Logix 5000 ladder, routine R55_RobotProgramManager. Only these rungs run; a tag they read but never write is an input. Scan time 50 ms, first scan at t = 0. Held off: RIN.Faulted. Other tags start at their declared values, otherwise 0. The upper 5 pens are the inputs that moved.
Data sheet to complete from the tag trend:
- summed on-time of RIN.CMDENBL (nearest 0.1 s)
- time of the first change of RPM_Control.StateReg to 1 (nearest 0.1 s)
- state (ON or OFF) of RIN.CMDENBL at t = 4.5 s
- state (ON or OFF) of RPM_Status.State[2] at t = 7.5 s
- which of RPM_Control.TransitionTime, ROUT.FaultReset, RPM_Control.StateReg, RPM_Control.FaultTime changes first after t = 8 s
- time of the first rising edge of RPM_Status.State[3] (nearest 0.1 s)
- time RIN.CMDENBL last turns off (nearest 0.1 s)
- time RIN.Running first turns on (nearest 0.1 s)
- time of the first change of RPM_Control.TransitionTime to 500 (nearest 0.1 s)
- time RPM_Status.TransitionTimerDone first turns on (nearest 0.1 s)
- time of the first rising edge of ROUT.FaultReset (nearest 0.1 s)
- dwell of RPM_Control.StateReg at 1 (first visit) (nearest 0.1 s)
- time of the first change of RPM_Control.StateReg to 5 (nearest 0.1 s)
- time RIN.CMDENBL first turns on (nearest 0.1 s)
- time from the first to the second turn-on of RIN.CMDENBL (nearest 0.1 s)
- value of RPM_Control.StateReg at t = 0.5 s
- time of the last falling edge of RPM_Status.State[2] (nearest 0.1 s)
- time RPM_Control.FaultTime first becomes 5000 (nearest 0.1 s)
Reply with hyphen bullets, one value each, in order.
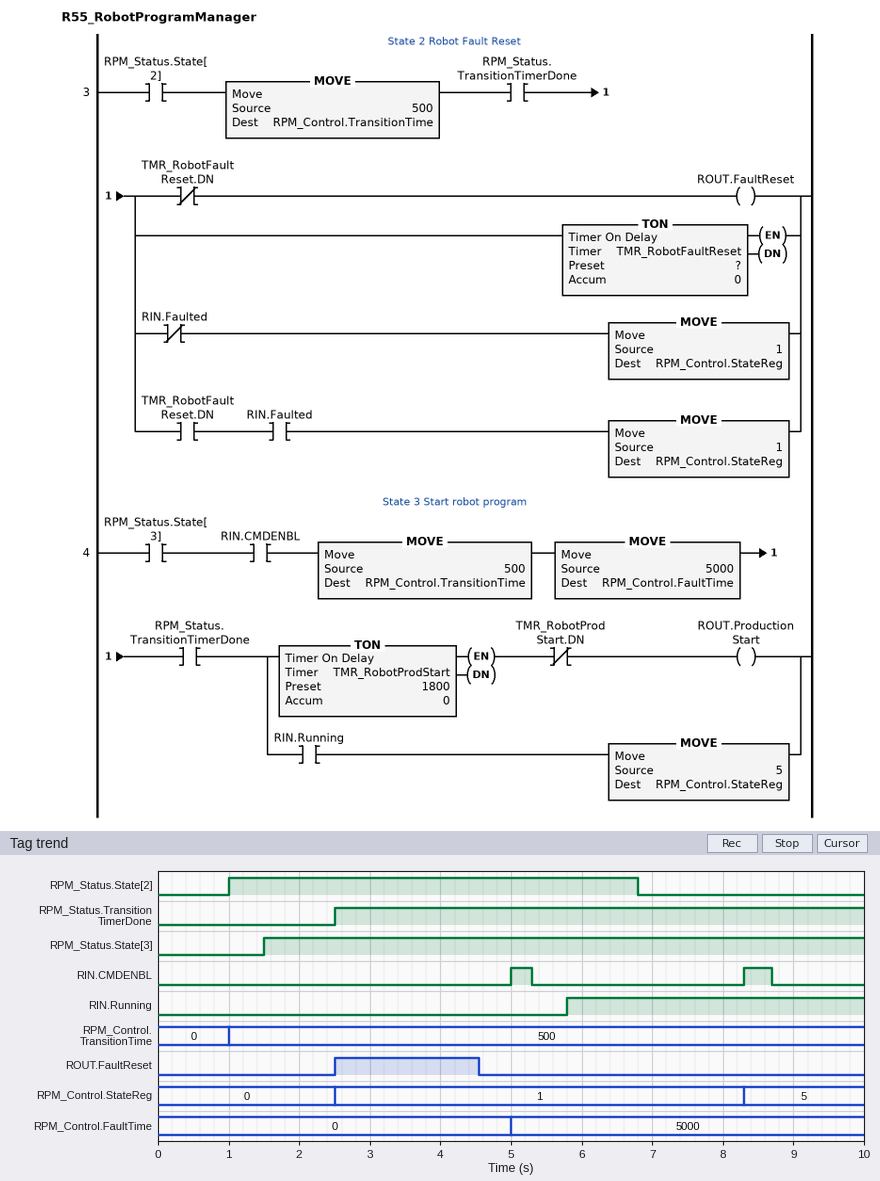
- 0.7 s
- 2.5 s
- OFF
- OFF
- RPM_Control.StateReg
- 1.5 s
- 8.7 s
- 5.8 s
- 1.0 s
- 2.5 s
- 2.5 s
- 5.8 s
- 8.3 s
- 5.0 s
- 3.3 s
- 0
- 6.8 s
- 5.0 s
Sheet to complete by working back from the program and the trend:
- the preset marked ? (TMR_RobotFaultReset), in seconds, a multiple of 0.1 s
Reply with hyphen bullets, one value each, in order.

- 2.0 s
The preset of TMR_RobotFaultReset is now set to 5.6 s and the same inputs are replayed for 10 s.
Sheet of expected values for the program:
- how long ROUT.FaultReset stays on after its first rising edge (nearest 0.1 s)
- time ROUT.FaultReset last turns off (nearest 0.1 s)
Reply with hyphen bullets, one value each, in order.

- 4.3 s
- 6.8 s
